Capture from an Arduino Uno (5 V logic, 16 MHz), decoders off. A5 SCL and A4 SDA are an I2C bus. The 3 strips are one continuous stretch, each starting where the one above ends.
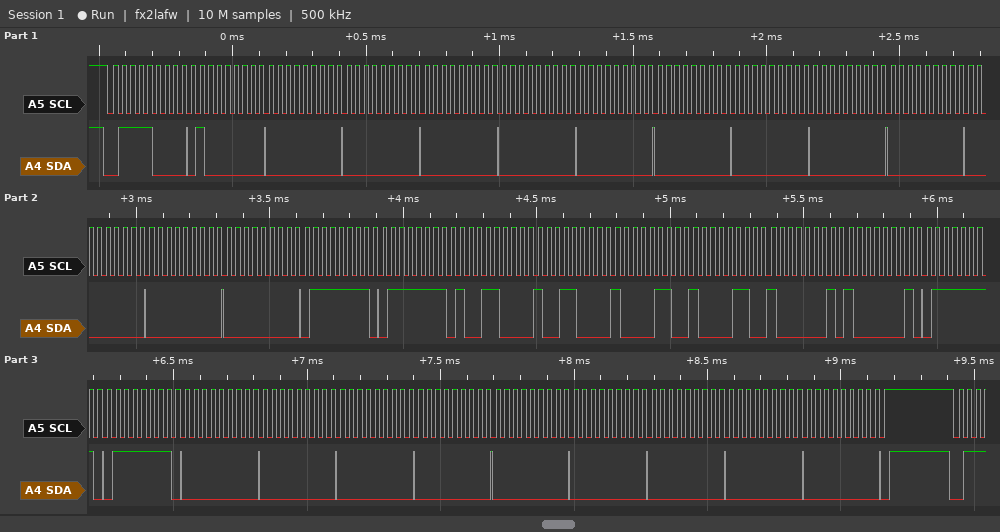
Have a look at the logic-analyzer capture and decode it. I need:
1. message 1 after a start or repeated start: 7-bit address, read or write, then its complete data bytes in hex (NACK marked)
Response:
0x3C write: 40 00 00 00 00 00 00 00 00 00 00 00 00 7F 7F 98 98 86 86 81 81 7F 7F 00 00 00 00 00 00 00 00 00
